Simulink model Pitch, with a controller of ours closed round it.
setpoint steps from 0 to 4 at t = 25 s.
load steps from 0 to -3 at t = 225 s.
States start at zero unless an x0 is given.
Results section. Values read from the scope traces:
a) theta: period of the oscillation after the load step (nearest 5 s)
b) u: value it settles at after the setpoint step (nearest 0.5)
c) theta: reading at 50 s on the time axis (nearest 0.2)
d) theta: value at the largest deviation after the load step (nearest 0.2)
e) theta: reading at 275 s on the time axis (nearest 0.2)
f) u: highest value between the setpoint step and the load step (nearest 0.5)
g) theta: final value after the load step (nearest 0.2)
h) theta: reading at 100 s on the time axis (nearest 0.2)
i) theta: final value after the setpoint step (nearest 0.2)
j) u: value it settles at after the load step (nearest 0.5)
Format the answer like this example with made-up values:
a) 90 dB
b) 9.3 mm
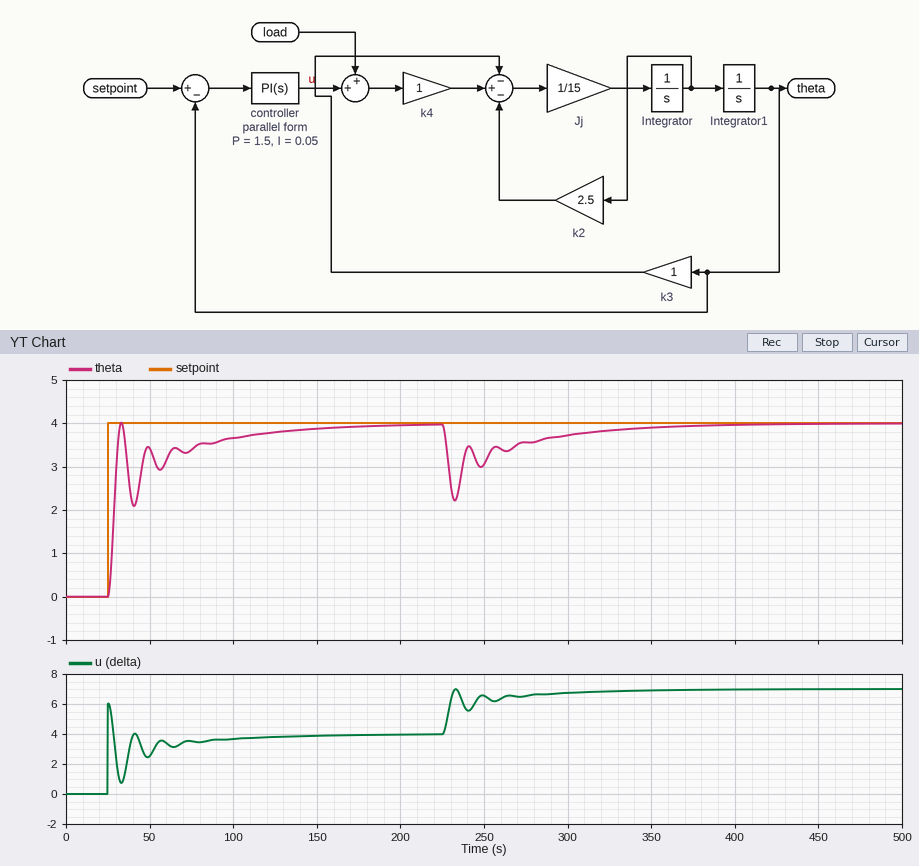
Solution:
a) 15 s
b) 4.0
c) 3.4
d) 2.2
e) 3.6
f) 6.0
g) 4.0
h) 3.6
i) 4.0
j) 7.0
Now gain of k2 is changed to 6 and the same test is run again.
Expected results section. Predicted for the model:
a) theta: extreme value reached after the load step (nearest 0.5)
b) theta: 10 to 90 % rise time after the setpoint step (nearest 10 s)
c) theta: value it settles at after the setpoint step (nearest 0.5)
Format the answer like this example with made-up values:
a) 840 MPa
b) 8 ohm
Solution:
a) 2.5
b) 60 s
c) 4.0
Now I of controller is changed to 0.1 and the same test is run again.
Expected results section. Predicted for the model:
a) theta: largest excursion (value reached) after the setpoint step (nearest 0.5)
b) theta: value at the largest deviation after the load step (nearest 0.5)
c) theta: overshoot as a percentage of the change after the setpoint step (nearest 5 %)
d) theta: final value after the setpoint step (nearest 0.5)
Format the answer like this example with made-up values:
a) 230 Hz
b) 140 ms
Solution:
a) 4.5
b) 2.5
c) 10 %
d) 4.0
